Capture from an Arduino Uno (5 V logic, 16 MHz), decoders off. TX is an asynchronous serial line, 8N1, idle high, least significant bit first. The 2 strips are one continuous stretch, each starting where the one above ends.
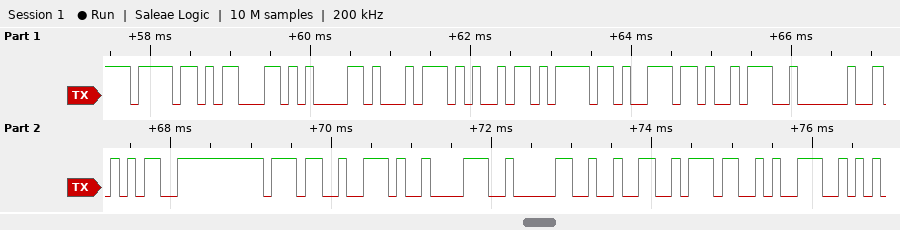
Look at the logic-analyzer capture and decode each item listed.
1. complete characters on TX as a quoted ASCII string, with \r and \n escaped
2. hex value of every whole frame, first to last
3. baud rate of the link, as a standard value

"ocation: 57.80279"
6F 63 61 74 69 6F 6E 3A 20 35 37 2E 38 30 32 37 39
9600 baud
